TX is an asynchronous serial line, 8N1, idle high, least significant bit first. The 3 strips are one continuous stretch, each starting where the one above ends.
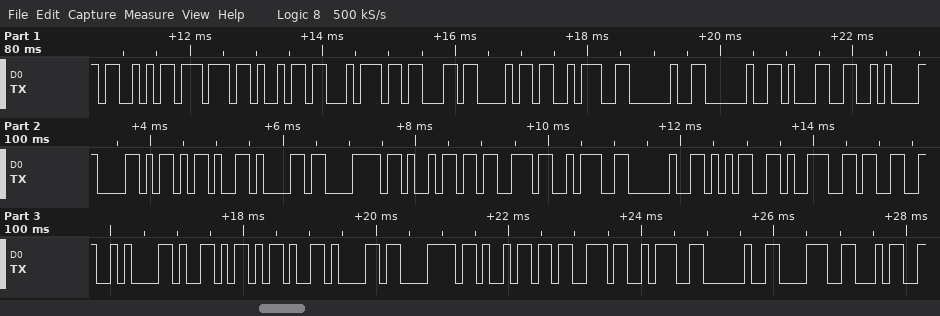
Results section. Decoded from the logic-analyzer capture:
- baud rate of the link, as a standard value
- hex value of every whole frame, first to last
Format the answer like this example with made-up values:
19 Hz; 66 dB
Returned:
9600 baud; 53 77 69 74 63 68 3A 20 20 31 0A 58 2D 61 78 69 73 3A 20 35 39 33 0A 59 2D 61 78 69 73 3A 20 38 34
